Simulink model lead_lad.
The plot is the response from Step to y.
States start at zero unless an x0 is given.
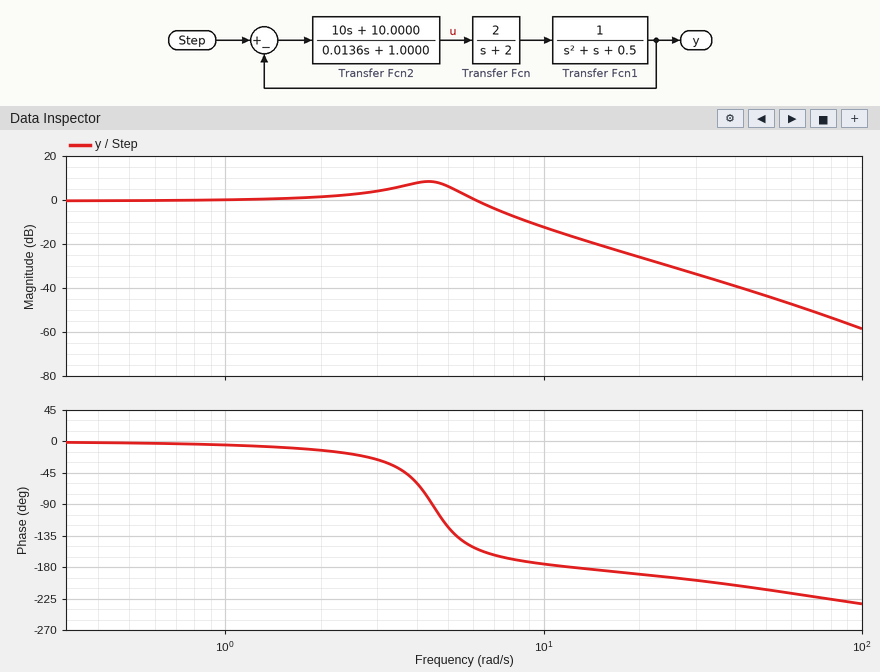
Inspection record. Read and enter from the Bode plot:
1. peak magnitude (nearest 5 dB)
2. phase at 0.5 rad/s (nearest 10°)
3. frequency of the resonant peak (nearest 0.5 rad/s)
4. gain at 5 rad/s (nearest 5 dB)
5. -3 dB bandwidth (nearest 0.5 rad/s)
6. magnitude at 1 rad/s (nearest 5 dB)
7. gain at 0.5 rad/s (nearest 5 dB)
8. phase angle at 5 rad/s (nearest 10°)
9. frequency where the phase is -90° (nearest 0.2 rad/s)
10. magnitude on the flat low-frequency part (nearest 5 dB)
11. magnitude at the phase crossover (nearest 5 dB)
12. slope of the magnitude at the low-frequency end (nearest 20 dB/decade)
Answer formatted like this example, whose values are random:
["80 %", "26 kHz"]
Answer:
["10 dB", "0°", "4.5 rad/s", "5 dB", "7.0 rad/s", "0 dB", "0 dB", "-120°", "4.4 rad/s", "0 dB", "-15 dB", "0 dB/decade"]
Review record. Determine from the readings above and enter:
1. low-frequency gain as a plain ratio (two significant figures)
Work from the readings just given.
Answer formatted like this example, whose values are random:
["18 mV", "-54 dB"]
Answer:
["1.0"]
